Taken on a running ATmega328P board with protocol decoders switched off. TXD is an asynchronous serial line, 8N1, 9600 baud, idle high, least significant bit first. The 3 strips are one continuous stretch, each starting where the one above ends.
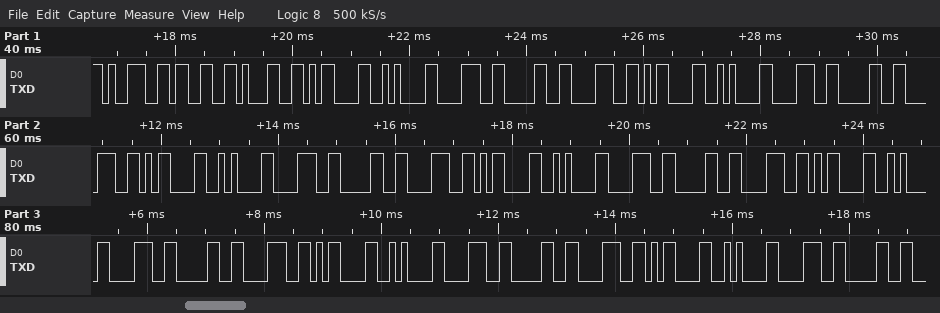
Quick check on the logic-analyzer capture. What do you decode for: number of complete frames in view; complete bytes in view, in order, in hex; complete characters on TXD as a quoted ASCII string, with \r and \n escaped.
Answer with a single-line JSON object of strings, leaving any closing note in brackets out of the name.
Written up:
{"number of complete frames in view": "37", "complete bytes in view, in order, in hex": "39 33 31 0D 0A 38 30 38 0D 0A 38 30 38 0D 0A 38 30 38 0D 0A 38 30 38 0D 0A 38 30 38 0D 0A 38 30 38 0D 0A 38 30", "complete characters on TXD as a quoted ASCII string, with \\r and \\n escaped": "\"931\\r\\n808\\r\\n808\\r\\n808\\r\\n808\\r\\n808\\r\\n808\\r\\n80\""}
